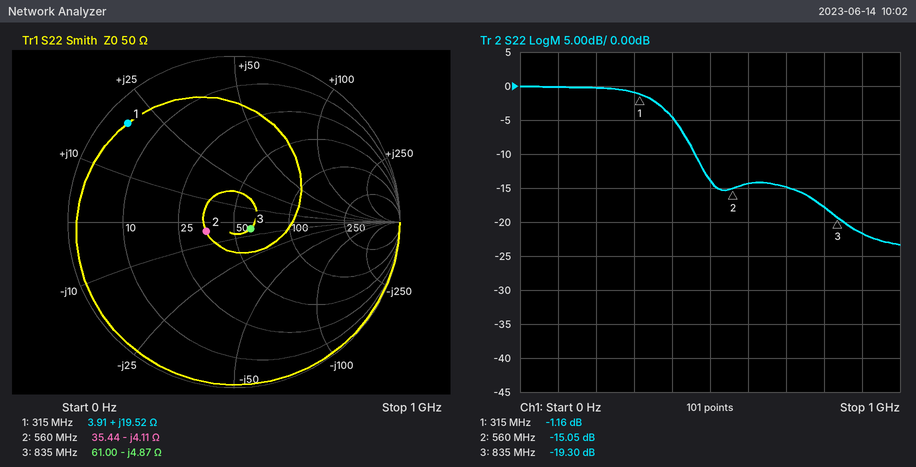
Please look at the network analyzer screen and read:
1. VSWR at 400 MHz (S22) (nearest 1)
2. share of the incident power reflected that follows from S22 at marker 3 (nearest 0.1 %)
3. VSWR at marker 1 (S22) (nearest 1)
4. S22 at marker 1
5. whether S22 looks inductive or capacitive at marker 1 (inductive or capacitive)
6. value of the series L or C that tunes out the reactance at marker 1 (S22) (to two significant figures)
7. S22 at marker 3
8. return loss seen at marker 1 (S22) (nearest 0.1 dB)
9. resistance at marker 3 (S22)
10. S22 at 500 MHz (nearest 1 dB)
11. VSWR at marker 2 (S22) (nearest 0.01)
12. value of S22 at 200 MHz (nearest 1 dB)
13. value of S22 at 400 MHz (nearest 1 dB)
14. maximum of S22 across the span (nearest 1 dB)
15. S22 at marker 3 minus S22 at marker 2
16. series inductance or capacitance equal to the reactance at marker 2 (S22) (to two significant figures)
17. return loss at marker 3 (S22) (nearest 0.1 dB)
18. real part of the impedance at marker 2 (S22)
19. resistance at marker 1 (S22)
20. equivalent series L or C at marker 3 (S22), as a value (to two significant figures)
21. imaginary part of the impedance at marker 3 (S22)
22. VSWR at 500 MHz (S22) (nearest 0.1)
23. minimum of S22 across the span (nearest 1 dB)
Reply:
4
1.2 %
15
-1.16 dB
inductive
26 pF
-19.30 dB
1.2 dB
61.00 Ω
-14 dB
1.43
0 dB
-5 dB
0 dB
-4.25 dB
69 pF
19.3 dB
35.44 Ω
3.91 Ω
39 pF
-4.87 Ω
1.5
-23 dB
